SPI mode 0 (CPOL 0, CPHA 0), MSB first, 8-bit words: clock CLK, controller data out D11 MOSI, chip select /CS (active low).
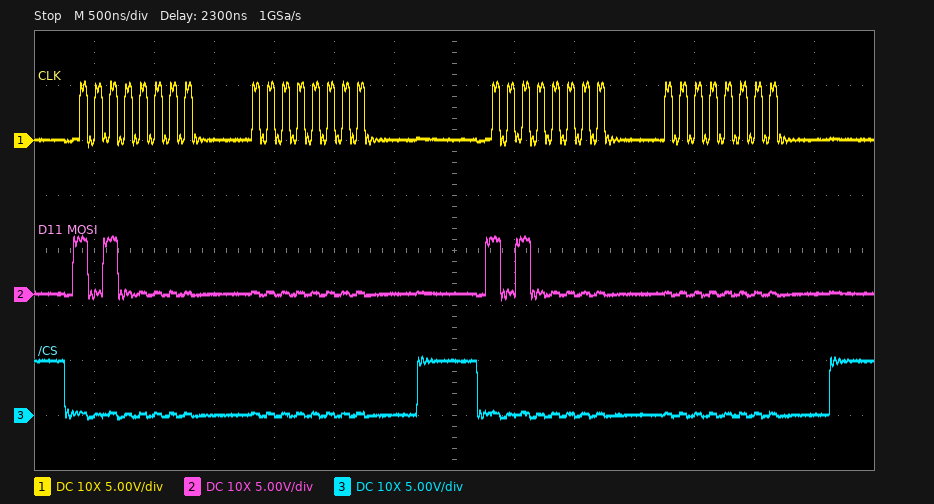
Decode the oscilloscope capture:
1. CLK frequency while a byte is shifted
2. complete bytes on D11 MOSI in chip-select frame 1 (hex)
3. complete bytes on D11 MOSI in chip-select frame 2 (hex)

8 MHz
A0 00
A0 00
